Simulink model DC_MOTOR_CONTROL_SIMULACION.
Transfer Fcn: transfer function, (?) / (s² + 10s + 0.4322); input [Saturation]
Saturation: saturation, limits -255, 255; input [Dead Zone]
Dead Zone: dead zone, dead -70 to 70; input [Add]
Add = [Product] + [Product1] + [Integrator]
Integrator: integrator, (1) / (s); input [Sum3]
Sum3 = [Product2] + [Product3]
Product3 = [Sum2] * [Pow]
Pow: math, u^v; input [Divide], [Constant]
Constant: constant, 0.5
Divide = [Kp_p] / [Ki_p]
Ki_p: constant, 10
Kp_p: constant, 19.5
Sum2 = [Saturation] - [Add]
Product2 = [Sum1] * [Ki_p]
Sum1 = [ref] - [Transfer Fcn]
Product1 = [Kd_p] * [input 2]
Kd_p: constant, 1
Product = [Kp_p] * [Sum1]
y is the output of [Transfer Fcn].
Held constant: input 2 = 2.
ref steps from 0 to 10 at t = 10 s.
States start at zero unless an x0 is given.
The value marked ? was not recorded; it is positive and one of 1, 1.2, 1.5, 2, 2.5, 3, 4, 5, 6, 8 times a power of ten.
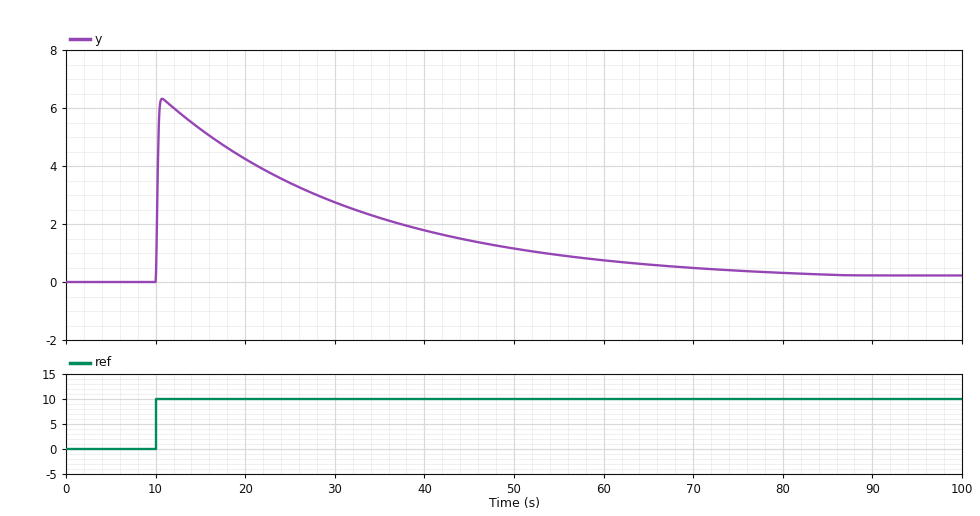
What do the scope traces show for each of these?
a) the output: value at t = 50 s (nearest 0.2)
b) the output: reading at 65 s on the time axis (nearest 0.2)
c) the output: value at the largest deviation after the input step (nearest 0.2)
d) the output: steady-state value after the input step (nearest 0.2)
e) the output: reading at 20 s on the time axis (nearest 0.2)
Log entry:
1.2
0.6
6.4
0.2
4.2
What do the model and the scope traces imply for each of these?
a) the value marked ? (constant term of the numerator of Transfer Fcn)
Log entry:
2.5
